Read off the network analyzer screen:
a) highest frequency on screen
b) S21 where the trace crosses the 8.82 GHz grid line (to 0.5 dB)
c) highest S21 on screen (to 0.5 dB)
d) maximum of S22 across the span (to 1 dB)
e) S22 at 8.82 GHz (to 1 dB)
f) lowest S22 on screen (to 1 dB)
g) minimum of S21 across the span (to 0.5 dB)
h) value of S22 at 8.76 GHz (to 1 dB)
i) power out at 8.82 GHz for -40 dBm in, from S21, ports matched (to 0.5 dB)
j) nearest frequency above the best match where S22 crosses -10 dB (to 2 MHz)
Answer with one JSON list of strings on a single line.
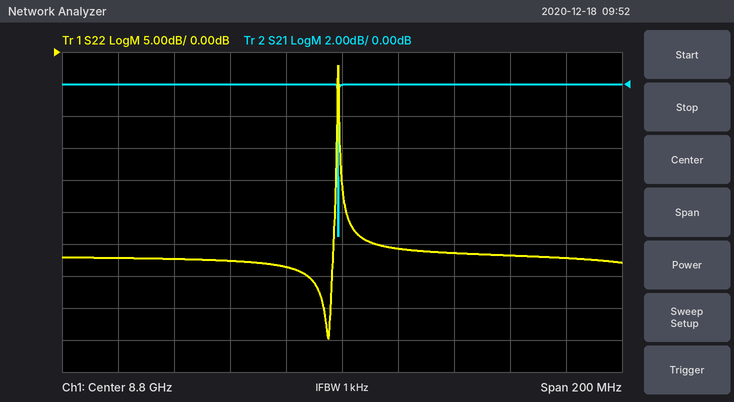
["8.9 GHz", "0.0 dB", "0.0 dB", "-2 dB", "-31 dB", "-45 dB", "-9.5 dB", "-33 dB", "-40.0 dBm", "8.798 GHz"]
